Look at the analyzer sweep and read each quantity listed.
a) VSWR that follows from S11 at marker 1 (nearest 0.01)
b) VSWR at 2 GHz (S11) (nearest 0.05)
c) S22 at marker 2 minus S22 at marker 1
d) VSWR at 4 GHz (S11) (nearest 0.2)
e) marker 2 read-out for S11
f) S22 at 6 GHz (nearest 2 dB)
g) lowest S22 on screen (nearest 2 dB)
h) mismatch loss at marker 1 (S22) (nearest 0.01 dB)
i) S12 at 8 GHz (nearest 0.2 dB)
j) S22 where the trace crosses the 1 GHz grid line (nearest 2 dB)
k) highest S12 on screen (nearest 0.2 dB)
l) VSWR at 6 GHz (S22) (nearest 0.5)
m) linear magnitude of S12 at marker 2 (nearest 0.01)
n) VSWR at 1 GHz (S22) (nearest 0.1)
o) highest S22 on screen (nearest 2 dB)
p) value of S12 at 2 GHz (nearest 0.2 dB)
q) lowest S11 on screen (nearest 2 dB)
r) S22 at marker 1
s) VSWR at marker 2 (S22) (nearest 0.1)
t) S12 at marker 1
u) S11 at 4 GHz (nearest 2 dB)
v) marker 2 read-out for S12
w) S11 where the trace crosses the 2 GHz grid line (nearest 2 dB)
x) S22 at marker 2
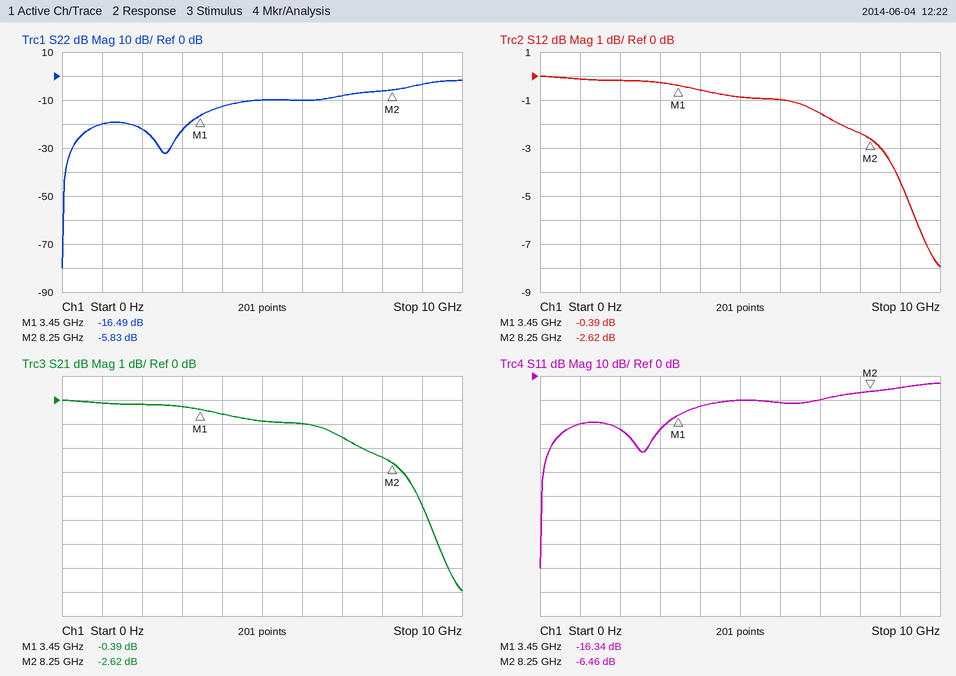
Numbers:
1.36
1.15
10.66 dB
1.6
-6.46 dB
-10 dB
-80 dB
0.10 dB
-2.4 dB
-20 dB
0.0 dB
2.0
0.74
1.2
-2 dB
-0.2 dB
-80 dB
-16.49 dB
3.1
-0.39 dB
-12 dB
-2.62 dB
-22 dB
-5.83 dB
